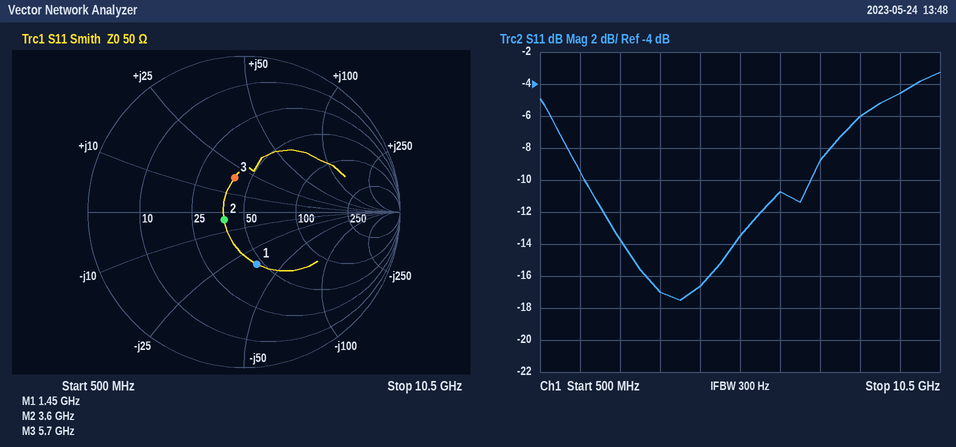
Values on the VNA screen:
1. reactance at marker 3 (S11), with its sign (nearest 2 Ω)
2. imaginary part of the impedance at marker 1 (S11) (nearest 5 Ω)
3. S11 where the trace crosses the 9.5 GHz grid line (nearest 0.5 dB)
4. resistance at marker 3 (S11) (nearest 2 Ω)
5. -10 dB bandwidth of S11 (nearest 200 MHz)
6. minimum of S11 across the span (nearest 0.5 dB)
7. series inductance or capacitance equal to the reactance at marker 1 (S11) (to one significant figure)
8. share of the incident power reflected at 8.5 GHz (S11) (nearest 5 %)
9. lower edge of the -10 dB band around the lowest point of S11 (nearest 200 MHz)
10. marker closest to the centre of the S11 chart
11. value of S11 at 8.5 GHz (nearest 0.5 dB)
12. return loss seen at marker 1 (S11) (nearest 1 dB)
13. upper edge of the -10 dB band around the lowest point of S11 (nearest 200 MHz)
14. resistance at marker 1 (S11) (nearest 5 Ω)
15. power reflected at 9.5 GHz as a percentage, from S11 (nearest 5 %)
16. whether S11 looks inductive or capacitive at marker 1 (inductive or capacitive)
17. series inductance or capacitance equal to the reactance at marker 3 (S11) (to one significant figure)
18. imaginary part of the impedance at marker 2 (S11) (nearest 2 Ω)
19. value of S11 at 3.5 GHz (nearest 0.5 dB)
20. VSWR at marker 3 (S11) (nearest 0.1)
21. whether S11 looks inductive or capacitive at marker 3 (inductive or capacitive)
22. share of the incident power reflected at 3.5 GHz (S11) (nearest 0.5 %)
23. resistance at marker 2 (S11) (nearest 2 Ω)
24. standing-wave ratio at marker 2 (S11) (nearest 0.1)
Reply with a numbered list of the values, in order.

1. +18 Ω
2. -35 Ω
3. -4.5 dB
4. 40 Ω
5. 5.6 GHz
6. -17.5 dB
7. 3 pF
8. 25 %
9. 1.6 GHz
10. marker 2
11. -6.0 dB
12. 9 dB
13. 7.2 GHz
14. 45 Ω
15. 35 %
16. capacitive
17. 500 pH
18. -4 Ω
19. -17.0 dB
20. 1.6
21. inductive
22. 2.0 %
23. 38 Ω
24. 1.3
